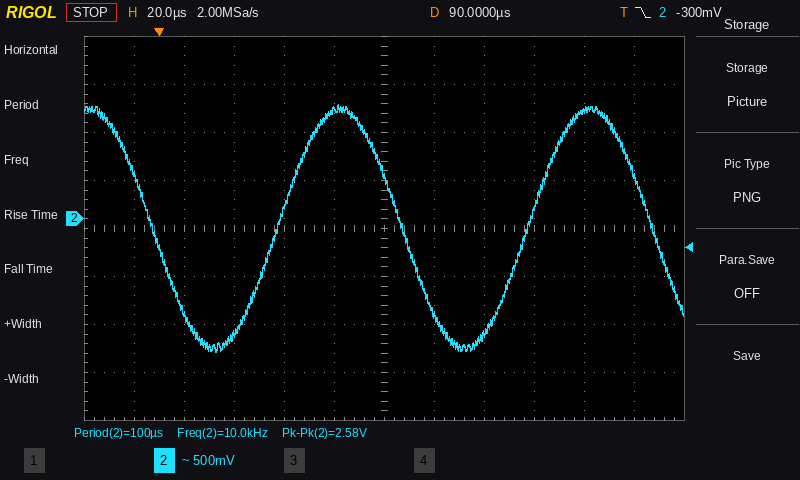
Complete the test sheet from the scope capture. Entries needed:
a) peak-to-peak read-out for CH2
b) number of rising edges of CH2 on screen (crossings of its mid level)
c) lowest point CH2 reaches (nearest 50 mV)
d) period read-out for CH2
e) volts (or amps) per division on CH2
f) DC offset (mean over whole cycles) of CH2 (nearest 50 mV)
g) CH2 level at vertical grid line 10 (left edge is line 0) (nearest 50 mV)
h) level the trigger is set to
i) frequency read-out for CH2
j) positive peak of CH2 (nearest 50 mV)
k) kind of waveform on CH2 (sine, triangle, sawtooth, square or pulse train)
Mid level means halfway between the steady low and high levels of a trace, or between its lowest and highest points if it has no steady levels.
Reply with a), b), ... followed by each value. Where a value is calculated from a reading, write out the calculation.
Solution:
a) 2.58 V
b) 2
c) -1.40 V
d) 100 µs
e) 500 mV
f) (1.20 V + (-1.40 V)) / 2 ≈ -100 mV
g) 1.15 V
h) -300 mV
i) 10.0 kHz
j) 1.20 V
k) sine
